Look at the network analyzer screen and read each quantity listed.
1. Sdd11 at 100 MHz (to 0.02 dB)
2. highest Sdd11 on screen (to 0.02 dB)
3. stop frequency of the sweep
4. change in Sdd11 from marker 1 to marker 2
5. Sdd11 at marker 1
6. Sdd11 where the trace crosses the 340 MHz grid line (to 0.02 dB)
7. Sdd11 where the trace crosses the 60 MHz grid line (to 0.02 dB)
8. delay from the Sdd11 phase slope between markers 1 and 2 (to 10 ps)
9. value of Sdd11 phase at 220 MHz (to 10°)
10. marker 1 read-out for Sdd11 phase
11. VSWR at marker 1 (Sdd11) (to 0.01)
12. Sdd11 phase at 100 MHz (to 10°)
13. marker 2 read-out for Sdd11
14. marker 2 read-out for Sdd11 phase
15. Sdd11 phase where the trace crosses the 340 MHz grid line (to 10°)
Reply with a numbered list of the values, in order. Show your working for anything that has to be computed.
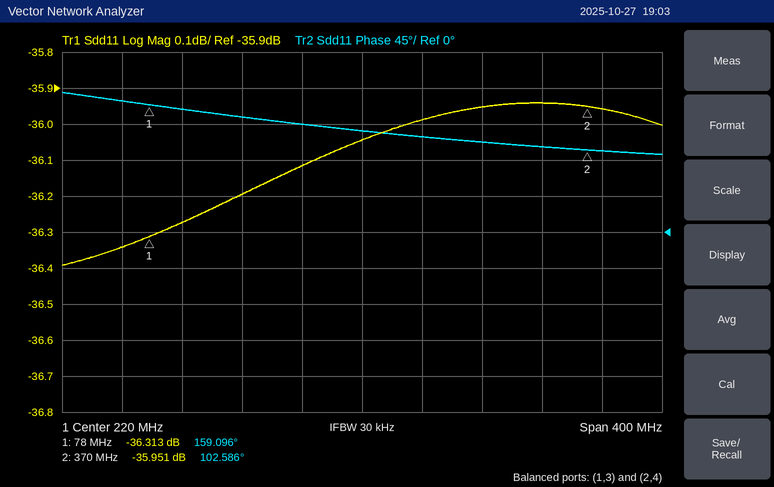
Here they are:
1. -36.28 dB
2. -35.94 dB
3. 420 MHz
4. -35.951 − (-36.313) = 0.362 dB
5. -36.313 dB
6. -35.94 dB
7. -36.34 dB
8. −(102.586° − (159.096°))/(360° × 292 MHz) ≈ 538 ps, so 540 ps to the nearest 10 ps
9. 130°
10. 159.096°
11. (1 + 0.0153)/(1 − 0.0153) ≈ 1.03
12. 150°
13. -35.951 dB
14. 102.586°
15. 110°
